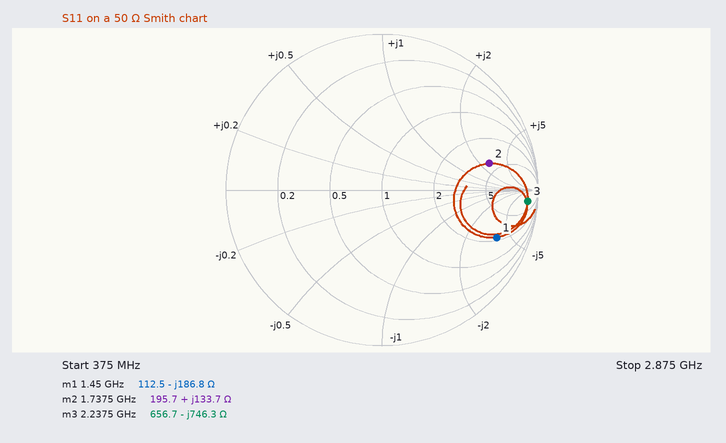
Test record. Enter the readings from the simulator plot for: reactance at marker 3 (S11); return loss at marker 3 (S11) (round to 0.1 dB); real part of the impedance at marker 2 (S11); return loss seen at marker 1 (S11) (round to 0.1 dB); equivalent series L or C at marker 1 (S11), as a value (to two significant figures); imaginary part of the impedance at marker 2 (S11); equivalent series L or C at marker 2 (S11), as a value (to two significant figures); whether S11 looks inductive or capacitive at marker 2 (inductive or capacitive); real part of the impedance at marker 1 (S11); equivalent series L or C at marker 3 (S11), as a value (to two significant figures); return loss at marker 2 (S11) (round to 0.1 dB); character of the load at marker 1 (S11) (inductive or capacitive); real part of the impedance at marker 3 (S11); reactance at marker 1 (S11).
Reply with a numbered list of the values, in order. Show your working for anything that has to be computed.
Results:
1. -746.3 Ω
2. 0.6 dB
3. 195.7 Ω
4. 2.0 dB
5. C = 1/(2π × 1.45 GHz × 186.8 Ω) ≈ 588 fF, so 590 fF to two significant figures
6. +133.7 Ω
7. L = 133.7 Ω/(2π × 1.7375 GHz) ≈ 12 nH
8. inductive
9. 112.5 Ω
10. C = 1/(2π × 2.2375 GHz × 746.3 Ω) ≈ 95 fF
11. 3.0 dB
12. capacitive
13. 656.7 Ω
14. -186.8 Ω
